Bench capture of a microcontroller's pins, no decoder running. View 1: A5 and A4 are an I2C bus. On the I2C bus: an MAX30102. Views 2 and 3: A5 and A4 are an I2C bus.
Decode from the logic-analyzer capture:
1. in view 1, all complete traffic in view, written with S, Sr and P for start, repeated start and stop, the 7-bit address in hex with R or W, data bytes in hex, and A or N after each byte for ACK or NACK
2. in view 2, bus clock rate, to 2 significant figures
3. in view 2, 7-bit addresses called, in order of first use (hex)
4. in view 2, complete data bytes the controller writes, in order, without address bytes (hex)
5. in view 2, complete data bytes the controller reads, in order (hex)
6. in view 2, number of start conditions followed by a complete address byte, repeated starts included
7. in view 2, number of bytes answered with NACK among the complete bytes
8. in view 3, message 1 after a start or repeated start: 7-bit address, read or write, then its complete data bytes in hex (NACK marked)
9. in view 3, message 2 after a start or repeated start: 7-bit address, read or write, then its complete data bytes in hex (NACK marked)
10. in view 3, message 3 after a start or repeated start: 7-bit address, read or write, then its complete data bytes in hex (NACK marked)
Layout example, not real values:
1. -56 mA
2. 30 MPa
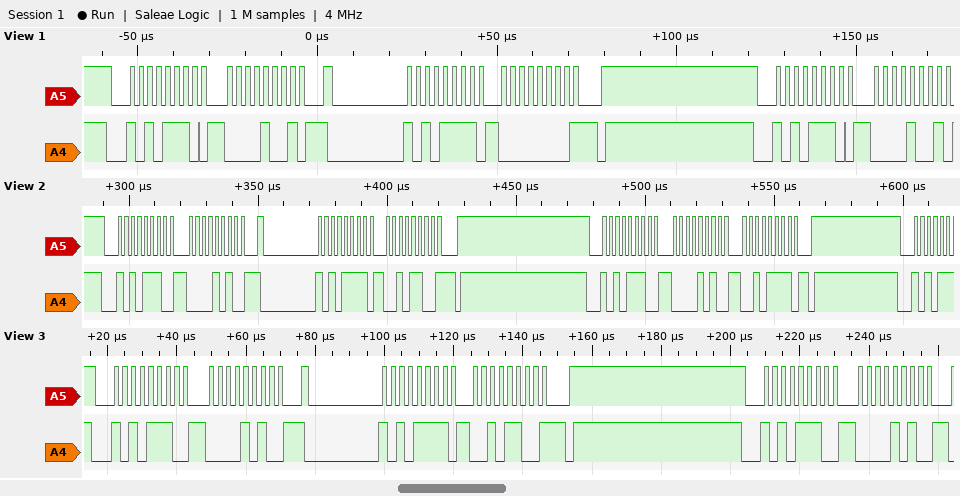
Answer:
1. S 57W A 09 A Sr 57R A 00 N P S 57W A 09 A
2. 400 kHz
3. 0x57
4. 0A 0A 2F
5. 2C
6. 3
7. 1
8. 0x57 write: 0A
9. 0x57 read: 2C NACK
10. 0x57 write: 0A
